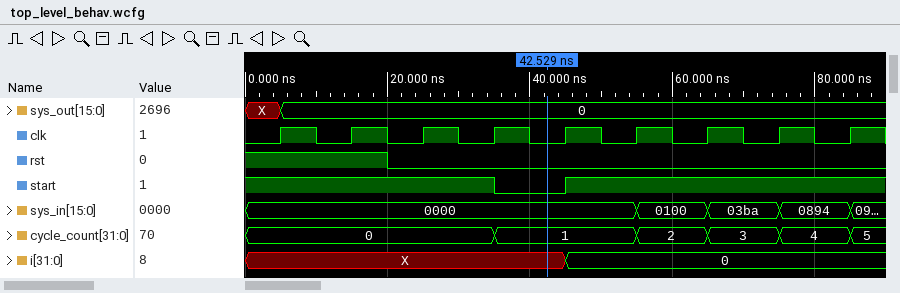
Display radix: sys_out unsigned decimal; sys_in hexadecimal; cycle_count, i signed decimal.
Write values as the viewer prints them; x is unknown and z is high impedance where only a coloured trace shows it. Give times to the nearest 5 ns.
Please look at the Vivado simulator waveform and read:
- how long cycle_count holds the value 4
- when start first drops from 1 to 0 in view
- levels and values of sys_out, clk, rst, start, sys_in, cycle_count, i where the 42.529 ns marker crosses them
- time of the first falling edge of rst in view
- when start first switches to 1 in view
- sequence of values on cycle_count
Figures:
10 ns
35 ns
sys_out=0, clk=0, rst=0, start=0, sys_in=0000, cycle_count=1, i=X
20 ns
45 ns
0, 1, 2, 3, 4, 5
